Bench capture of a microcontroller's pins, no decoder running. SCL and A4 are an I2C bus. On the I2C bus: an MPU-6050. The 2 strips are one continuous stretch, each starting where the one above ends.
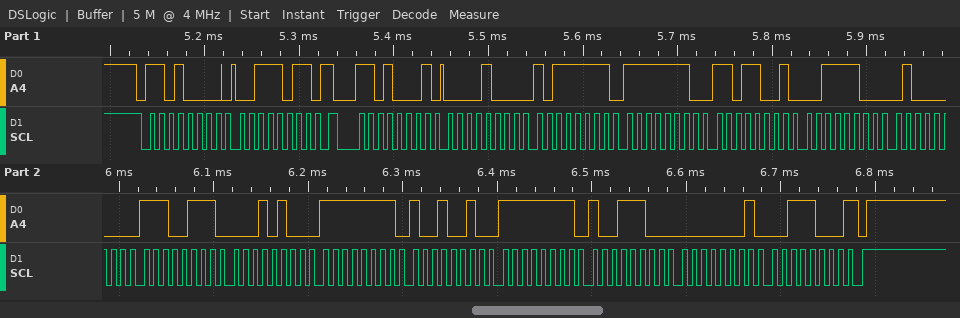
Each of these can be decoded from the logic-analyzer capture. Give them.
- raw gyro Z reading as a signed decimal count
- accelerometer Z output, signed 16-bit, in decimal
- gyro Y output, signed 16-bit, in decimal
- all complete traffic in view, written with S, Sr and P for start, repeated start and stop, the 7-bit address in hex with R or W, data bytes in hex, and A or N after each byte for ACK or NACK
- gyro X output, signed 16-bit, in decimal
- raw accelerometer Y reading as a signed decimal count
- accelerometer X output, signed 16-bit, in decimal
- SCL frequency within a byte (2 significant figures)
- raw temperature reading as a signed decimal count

312
15424
-100
S 68W A 3B A Sr 68R A 08 A BF A FE A D9 A 3C A 40 A E7 A 14 A FF A 92 A FF A 9C A 01 A 38 N P
-110
-295
2239
100 kHz
-6380
